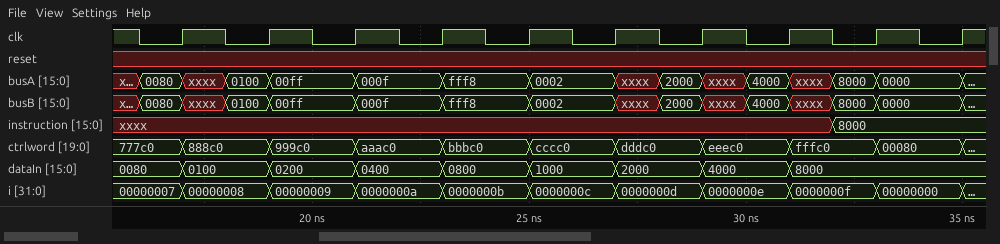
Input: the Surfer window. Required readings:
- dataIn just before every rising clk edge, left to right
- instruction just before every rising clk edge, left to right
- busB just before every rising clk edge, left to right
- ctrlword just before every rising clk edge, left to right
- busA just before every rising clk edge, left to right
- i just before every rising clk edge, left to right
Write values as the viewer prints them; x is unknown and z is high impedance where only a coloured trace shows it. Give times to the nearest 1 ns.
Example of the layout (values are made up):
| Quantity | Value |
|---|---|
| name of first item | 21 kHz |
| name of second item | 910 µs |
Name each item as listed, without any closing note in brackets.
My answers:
| Quantity | Value |
|---|---|
| dataIn just before every rising clk edge, left to right | 0080, 0100, 0200, 0400, 0800, 1000, 2000, 4000, 8000, 8000 |
| instruction just before every rising clk edge, left to right | xxxx, xxxx, xxxx, xxxx, xxxx, xxxx, xxxx, xxxx, 8000, 8000 |
| busB just before every rising clk edge, left to right | 0080, 0100, 00ff, 000f, fff8, 0002, 2000, 4000, 8000, 0000 |
| ctrlword just before every rising clk edge, left to right | 777c0, 888c0, 999c0, aaac0, bbbc0, cccc0, dddc0, eeec0, fffc0, 00080 |
| busA just before every rising clk edge, left to right | 0080, 0100, 00ff, 000f, fff8, 0002, 2000, 4000, 8000, 0000 |
| i just before every rising clk edge, left to right | 00000007, 00000008, 00000009, 0000000a, 0000000b, 0000000c, 0000000d, 0000000e, 0000000f, 00000000 |
